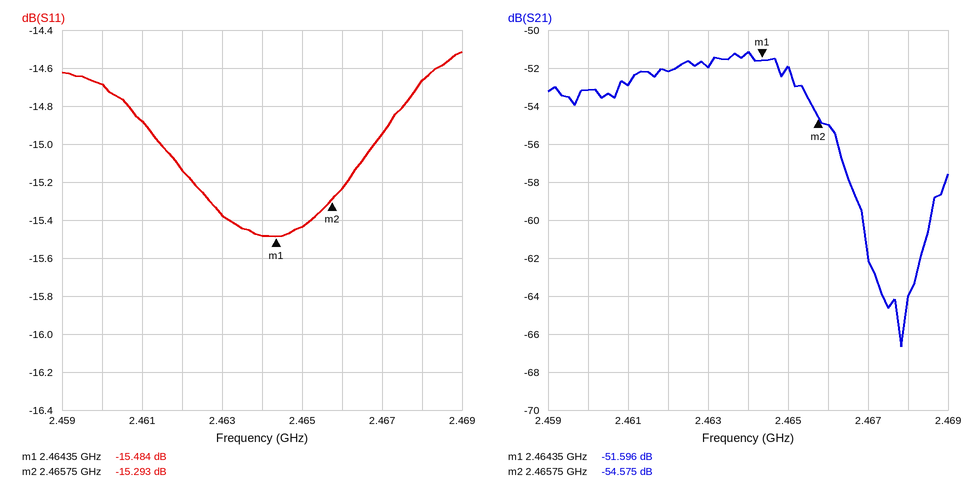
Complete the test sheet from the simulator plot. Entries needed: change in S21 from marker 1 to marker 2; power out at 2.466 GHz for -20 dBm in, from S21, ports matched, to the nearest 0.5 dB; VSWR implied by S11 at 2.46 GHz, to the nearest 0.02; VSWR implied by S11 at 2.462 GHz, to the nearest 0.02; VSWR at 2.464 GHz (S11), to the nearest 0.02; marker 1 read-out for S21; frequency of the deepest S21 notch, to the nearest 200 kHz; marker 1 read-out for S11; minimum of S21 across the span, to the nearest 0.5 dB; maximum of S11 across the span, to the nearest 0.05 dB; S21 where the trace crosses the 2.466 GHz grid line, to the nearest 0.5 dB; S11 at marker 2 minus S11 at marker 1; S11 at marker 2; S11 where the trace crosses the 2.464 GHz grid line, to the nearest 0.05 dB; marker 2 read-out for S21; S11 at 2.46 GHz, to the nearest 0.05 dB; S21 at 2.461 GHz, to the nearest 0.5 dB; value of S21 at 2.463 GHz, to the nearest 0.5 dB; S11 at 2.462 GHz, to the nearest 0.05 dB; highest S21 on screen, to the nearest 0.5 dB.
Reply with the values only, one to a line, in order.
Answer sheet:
-2.979 dB
-75.0 dBm
1.46
1.42
1.40
-51.596 dB
2.4678 GHz
-15.484 dB
-66.5 dB
-14.50 dB
-55.0 dB
0.191 dB
-15.293 dB
-15.50 dB
-54.575 dB
-14.70 dB
-53.0 dB
-52.0 dB
-15.15 dB
-51.0 dB
